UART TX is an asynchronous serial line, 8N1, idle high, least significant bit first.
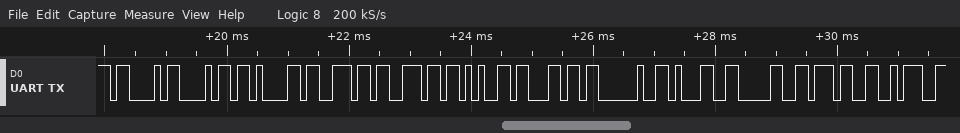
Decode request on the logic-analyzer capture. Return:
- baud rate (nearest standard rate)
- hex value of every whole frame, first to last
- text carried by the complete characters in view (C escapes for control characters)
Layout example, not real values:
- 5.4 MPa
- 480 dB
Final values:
- 9600 baud
- 0x43 0x68 0x61 0x6E 0x6E 0x65 0x6C 0x20 0x31 0x30 0x37 0x3A
- "Channel 107:"
